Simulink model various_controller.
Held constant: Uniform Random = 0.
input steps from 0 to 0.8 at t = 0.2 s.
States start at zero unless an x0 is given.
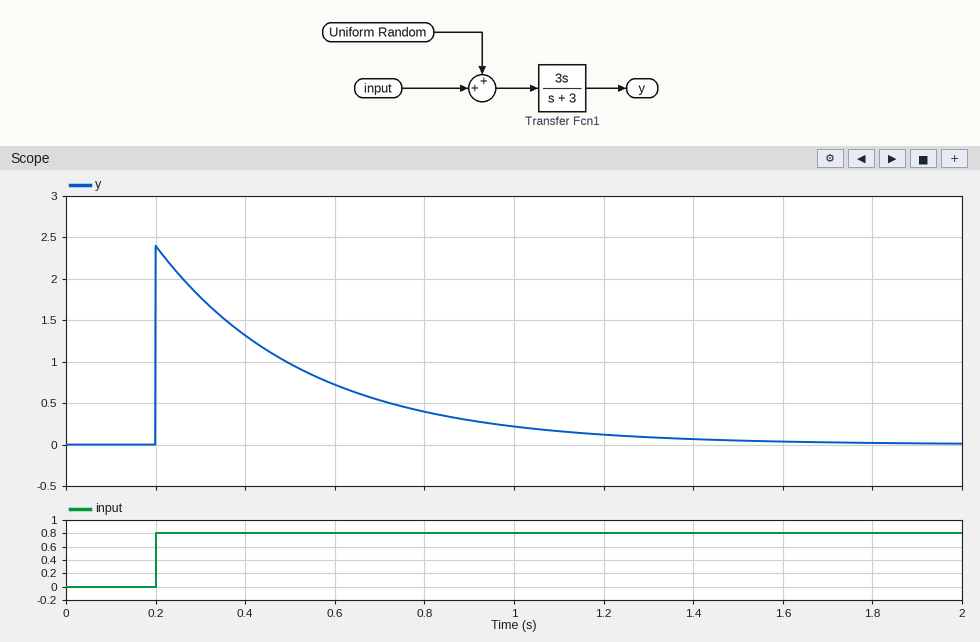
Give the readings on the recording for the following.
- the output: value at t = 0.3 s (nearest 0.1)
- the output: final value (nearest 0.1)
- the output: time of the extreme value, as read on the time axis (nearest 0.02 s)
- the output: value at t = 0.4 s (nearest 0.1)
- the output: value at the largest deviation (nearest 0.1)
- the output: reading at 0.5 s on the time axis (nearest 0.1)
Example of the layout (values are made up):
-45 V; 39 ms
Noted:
1.8; 0.0; 0.20 s; 1.3; 2.4; 1.0
